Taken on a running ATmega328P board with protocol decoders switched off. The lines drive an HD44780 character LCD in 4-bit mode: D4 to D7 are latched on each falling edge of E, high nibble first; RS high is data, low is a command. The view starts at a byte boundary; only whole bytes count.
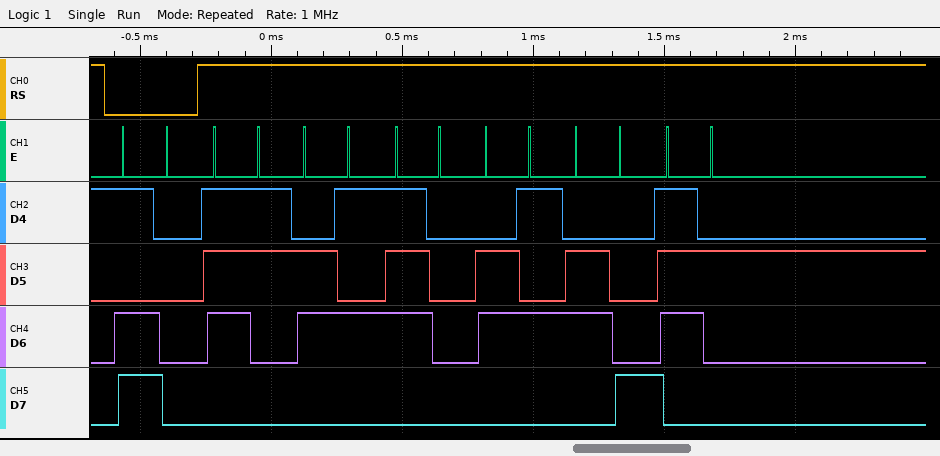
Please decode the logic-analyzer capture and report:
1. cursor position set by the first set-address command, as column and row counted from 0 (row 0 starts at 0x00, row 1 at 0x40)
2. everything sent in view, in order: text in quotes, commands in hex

column 16, row 1
0xD0 "sepehr"
